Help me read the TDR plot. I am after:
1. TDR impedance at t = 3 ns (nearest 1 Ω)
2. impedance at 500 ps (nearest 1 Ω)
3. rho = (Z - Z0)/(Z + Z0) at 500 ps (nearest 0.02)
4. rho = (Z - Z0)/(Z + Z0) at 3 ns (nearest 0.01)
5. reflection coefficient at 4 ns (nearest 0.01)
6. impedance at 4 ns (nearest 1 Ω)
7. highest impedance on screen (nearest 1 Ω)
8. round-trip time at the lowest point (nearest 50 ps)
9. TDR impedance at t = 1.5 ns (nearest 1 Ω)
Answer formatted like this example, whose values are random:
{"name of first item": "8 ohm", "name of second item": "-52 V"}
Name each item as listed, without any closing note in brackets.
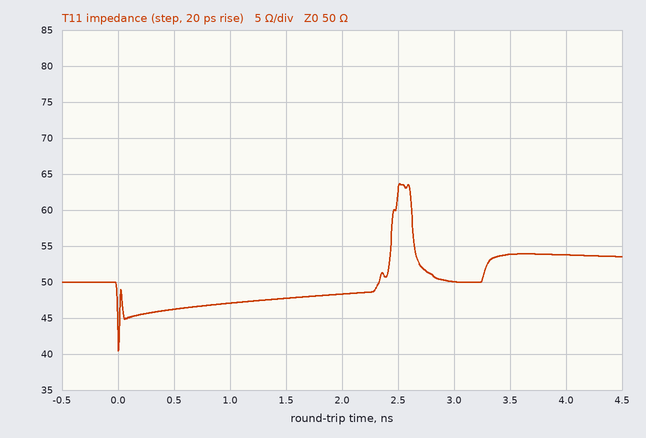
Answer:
{"TDR impedance at t = 3 ns": "50 Ω", "impedance at 500 ps": "46 Ω", "rho = (Z - Z0)/(Z + Z0) at 500 ps": "-0.04", "rho = (Z - Z0)/(Z + Z0) at 3 ns": "0.00", "reflection coefficient at 4 ns": "+0.04", "impedance at 4 ns": "54 Ω", "highest impedance on screen": "64 Ω", "round-trip time at the lowest point": "0 ps", "TDR impedance at t = 1.5 ns": "48 Ω"}
